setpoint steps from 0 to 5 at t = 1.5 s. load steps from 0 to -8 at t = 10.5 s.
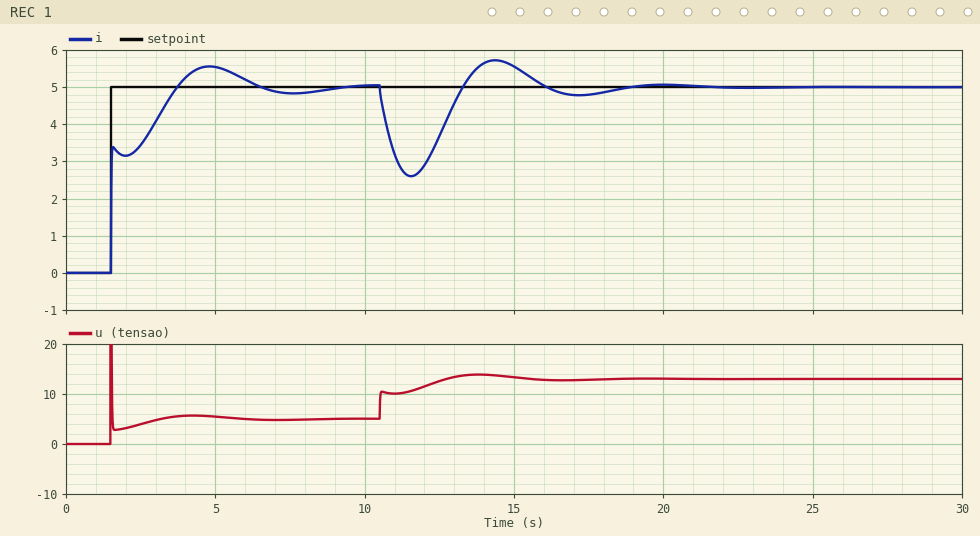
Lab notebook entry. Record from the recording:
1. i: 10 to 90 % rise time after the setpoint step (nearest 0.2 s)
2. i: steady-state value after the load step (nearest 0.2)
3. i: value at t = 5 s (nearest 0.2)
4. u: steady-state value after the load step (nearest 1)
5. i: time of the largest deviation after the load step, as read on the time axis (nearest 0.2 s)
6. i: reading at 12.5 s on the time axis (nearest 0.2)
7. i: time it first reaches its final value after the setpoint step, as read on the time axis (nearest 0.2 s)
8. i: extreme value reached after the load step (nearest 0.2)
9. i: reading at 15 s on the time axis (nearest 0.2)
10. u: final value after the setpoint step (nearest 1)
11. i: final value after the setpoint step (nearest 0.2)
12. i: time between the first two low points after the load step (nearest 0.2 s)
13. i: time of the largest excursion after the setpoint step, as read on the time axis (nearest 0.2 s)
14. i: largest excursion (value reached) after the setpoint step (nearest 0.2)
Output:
1.8 s
5.0
5.6
13
11.6 s
3.6
3.8 s
2.6
5.6
5
5.0
5.6 s
4.8 s
5.6
